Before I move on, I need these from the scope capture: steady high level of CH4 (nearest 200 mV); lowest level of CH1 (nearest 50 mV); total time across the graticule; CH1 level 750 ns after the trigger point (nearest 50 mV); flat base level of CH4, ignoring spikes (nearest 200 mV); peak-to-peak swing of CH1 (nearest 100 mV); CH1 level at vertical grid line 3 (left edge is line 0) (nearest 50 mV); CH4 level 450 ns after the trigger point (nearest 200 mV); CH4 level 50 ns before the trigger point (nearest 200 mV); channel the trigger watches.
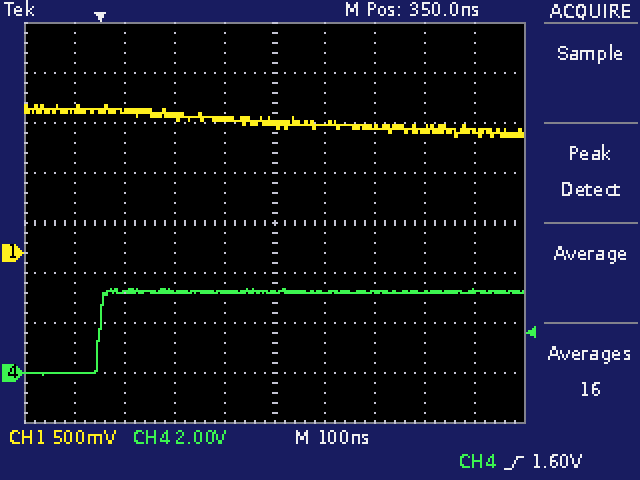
3.2 V
1.15 V
1 µs
1.20 V
0.0 V
300 mV
1.35 V
3.2 V
0.0 V
CH4
